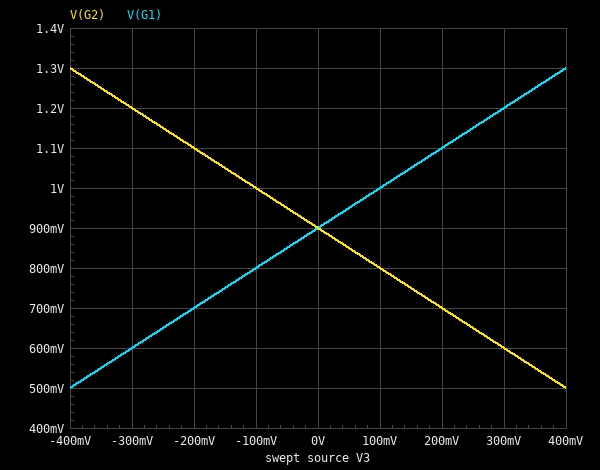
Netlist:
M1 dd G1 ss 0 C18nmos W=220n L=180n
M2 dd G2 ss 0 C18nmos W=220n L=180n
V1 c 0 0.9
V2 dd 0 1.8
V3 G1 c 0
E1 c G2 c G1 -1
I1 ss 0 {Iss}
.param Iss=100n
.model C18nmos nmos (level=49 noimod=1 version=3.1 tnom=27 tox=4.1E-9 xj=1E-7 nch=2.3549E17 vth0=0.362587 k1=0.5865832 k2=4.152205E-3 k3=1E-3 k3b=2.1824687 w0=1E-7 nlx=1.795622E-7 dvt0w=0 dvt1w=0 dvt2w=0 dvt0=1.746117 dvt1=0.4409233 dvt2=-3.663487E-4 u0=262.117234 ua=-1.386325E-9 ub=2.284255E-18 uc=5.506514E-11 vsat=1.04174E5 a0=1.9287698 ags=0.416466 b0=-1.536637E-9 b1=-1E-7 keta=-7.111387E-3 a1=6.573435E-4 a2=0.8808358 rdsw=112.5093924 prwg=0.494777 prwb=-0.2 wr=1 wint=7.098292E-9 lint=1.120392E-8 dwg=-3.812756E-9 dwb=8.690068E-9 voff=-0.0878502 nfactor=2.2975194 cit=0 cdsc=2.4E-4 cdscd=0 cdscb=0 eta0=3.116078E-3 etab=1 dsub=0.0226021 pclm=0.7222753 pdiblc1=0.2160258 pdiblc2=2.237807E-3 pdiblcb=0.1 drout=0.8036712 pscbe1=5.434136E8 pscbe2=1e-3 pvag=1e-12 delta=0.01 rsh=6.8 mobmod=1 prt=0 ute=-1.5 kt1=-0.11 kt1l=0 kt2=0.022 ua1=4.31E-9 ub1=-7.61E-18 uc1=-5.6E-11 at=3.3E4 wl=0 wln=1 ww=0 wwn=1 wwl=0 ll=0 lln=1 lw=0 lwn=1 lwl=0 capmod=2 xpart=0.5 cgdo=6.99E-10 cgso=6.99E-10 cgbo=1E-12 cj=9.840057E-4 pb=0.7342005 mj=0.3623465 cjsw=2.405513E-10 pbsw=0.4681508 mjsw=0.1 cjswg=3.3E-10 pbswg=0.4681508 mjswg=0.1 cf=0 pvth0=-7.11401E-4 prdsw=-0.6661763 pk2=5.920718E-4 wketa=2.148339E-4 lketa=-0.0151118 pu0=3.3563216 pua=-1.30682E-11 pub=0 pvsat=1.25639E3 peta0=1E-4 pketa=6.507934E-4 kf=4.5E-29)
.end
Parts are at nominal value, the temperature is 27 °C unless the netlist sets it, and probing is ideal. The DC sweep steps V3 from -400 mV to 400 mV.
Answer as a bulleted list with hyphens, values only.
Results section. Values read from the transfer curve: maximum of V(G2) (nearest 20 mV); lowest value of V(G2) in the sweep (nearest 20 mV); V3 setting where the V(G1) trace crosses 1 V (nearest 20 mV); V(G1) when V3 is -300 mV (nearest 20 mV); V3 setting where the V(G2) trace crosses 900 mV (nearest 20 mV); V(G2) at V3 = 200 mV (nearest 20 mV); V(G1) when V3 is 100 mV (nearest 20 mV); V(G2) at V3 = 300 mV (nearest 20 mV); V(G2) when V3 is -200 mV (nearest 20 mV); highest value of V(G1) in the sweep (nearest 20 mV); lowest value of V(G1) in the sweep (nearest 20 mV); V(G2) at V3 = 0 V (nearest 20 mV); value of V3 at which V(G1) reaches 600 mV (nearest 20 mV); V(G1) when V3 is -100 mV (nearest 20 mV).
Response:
- 1.30 V
- 500 mV
- 100 mV
- 600 mV
- 0 V
- 700 mV
- 1.00 V
- 600 mV
- 1.10 V
- 1.30 V
- 500 mV
- 900 mV
- -300 mV
- 800 mV
